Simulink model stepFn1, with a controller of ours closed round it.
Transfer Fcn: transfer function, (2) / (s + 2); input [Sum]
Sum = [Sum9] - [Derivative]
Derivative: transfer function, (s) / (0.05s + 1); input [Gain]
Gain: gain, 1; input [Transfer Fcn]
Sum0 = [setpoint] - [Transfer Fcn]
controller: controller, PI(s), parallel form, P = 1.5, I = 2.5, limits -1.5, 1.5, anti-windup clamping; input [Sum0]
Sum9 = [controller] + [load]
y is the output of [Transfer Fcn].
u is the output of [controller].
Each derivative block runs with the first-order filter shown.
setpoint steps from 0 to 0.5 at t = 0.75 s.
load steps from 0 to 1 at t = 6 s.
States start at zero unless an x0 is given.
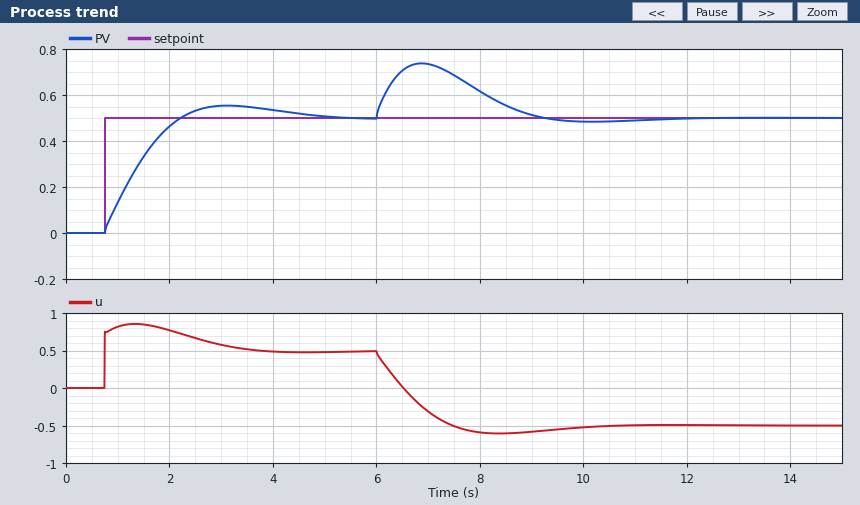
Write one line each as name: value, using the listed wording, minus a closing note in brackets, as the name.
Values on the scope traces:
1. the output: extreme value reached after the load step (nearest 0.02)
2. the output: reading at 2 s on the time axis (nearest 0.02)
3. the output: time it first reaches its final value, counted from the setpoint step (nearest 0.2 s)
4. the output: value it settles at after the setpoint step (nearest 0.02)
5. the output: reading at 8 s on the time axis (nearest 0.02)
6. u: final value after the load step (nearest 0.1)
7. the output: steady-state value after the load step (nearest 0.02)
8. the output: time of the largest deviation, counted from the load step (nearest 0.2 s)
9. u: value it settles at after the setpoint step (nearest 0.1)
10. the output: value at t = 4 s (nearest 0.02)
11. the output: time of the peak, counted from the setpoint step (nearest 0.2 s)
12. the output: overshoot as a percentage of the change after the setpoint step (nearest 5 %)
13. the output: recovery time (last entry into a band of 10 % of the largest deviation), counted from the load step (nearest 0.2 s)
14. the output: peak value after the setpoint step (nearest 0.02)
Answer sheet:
the output: extreme value reached after the load step: 0.74
the output: reading at 2 s on the time axis: 0.46
the output: time it first reaches its final value, counted from the setpoint step: 1.4 s
the output: value it settles at after the setpoint step: 0.50
the output: reading at 8 s on the time axis: 0.62
u: final value after the load step: -0.5
the output: steady-state value after the load step: 0.50
the output: time of the largest deviation, counted from the load step: 0.8 s
u: value it settles at after the setpoint step: 0.5
the output: value at t = 4 s: 0.54
the output: time of the peak, counted from the setpoint step: 2.4 s
the output: overshoot as a percentage of the change after the setpoint step: 10 %
the output: recovery time (last entry into a band of 10 % of the largest deviation), counted from the load step: 2.8 s
the output: peak value after the setpoint step: 0.56
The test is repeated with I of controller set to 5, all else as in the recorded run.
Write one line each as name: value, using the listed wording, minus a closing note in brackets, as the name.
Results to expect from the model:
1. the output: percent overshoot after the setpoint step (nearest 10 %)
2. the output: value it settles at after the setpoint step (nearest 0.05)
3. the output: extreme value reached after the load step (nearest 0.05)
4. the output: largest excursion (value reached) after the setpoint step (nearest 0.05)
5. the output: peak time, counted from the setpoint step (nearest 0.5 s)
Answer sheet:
the output: percent overshoot after the setpoint step: 20 %
the output: value it settles at after the setpoint step: 0.50
the output: extreme value reached after the load step: 0.70
the output: largest excursion (value reached) after the setpoint step: 0.60
the output: peak time, counted from the setpoint step: 1.5 s
